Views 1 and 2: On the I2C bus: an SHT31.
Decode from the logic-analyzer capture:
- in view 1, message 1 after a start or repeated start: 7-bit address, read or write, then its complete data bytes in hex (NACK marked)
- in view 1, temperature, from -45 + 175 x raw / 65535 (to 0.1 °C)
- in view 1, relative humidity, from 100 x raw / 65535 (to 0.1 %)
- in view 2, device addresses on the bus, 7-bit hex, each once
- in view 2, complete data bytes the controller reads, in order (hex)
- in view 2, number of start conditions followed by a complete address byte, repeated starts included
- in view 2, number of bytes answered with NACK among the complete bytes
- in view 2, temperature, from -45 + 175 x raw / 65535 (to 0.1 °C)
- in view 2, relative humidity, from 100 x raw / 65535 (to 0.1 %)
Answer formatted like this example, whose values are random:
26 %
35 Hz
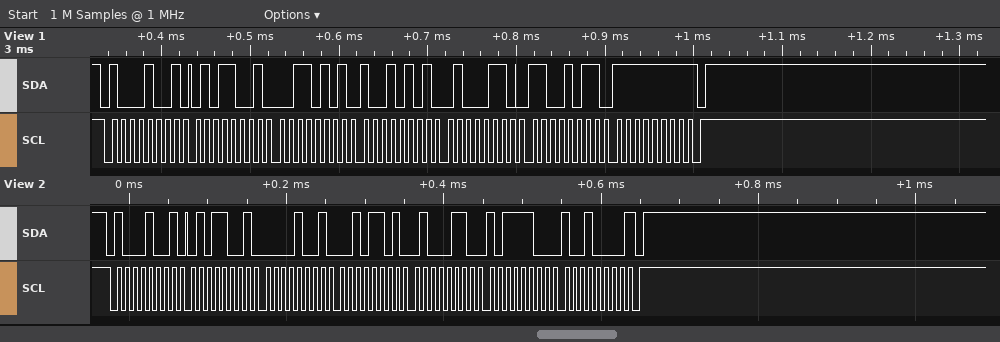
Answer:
0x44 read: 59 35 95 46 CB FF NACK
16.0 °C
27.7 %
0x44
59 09 2D 46 BC 90
1
1
15.9 °C
27.6 %
